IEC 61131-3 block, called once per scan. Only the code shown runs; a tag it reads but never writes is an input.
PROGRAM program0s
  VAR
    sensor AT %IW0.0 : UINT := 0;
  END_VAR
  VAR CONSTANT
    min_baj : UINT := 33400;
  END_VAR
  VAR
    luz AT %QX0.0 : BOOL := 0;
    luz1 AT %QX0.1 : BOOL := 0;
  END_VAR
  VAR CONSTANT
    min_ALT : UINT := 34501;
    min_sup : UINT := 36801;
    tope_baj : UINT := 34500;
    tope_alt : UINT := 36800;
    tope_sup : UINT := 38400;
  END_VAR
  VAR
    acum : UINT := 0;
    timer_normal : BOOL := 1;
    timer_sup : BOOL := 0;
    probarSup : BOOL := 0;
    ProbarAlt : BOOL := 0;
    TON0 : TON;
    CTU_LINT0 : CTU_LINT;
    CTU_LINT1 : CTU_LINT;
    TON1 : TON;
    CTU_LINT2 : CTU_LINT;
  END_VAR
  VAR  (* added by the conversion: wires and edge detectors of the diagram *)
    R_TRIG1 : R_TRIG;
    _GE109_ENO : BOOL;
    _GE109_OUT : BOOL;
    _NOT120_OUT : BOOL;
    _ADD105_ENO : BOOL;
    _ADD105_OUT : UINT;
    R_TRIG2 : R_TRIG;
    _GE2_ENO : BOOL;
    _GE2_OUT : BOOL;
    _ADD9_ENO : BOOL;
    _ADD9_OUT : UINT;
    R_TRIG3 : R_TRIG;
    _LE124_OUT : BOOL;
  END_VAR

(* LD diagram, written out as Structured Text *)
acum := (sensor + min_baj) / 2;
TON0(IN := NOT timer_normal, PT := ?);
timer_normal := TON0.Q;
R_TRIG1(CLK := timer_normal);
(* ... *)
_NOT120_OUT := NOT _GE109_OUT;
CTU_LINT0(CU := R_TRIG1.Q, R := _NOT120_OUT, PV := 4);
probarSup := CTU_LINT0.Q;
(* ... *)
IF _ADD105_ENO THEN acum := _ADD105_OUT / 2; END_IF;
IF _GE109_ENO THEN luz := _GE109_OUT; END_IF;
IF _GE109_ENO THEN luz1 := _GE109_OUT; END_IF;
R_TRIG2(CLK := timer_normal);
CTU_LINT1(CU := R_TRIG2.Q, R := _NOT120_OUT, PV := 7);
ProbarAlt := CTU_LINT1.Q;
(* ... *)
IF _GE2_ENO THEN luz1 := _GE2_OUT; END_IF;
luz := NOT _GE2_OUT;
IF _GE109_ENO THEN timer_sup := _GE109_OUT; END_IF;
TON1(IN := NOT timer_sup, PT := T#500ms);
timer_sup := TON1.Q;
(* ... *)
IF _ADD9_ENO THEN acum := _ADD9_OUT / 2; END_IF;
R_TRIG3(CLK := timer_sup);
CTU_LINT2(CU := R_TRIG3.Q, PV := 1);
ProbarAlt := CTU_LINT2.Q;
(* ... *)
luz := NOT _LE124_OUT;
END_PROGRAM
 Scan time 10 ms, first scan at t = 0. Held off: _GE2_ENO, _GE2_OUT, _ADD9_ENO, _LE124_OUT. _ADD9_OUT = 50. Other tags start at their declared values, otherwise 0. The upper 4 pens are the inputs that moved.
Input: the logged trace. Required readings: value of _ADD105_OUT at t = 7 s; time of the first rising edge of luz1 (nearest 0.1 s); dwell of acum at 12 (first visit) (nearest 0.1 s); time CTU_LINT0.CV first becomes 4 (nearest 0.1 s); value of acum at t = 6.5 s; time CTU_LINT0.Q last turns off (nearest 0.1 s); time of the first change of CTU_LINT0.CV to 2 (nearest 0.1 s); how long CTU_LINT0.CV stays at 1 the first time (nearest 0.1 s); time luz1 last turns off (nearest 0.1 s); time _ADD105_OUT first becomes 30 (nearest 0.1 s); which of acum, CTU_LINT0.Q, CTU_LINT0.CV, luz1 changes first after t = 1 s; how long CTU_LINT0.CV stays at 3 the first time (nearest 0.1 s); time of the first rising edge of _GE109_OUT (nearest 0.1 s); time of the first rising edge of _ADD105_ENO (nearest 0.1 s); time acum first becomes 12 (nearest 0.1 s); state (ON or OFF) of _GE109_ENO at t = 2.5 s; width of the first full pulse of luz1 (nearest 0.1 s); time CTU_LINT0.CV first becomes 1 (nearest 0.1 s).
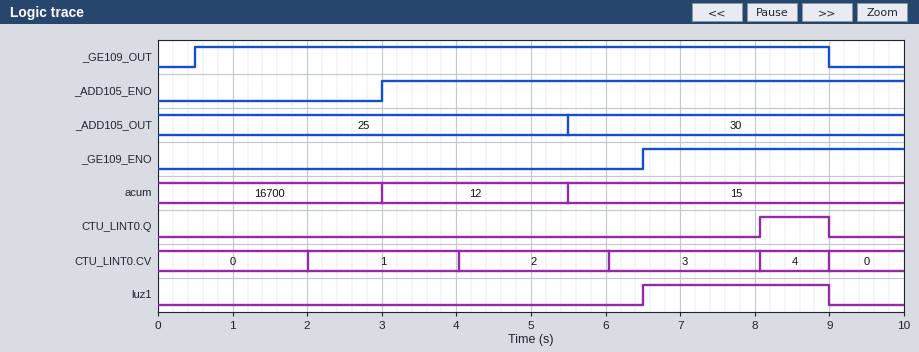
30
6.5 s
2.5 s
8.1 s
15
9.0 s
4.0 s
2.0 s
9.0 s
5.5 s
CTU_LINT0.CV
2.0 s
0.5 s
3.0 s
3.0 s
OFF
2.5 s
2.0 s
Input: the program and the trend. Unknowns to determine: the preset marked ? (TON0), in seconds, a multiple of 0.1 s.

2.0 s
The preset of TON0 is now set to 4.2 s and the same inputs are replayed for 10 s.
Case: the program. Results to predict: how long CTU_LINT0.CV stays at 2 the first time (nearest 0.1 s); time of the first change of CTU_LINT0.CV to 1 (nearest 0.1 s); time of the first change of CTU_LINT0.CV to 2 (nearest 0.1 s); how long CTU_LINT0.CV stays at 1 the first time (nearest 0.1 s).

0.6 s
4.2 s
8.4 s
4.2 s
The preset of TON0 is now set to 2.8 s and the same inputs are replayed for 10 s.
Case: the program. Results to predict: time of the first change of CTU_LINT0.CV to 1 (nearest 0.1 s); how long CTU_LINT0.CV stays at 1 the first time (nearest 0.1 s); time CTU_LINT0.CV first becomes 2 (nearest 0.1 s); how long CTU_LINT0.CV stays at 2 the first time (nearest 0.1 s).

2.8 s
2.8 s
5.6 s
2.8 s
